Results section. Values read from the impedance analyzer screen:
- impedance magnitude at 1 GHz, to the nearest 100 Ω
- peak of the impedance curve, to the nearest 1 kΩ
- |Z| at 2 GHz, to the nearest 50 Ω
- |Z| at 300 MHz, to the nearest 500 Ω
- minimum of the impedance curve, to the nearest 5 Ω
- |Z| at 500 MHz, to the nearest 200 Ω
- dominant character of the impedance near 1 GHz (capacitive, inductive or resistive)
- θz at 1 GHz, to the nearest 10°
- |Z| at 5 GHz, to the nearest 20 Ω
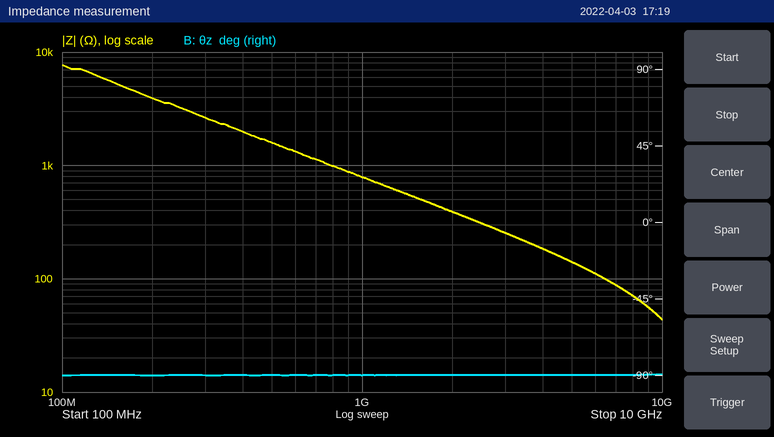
800 Ω
8 kΩ
400 Ω
2.5 kΩ
45 Ω
1.6 kΩ
capacitive
-90°
140 Ω
